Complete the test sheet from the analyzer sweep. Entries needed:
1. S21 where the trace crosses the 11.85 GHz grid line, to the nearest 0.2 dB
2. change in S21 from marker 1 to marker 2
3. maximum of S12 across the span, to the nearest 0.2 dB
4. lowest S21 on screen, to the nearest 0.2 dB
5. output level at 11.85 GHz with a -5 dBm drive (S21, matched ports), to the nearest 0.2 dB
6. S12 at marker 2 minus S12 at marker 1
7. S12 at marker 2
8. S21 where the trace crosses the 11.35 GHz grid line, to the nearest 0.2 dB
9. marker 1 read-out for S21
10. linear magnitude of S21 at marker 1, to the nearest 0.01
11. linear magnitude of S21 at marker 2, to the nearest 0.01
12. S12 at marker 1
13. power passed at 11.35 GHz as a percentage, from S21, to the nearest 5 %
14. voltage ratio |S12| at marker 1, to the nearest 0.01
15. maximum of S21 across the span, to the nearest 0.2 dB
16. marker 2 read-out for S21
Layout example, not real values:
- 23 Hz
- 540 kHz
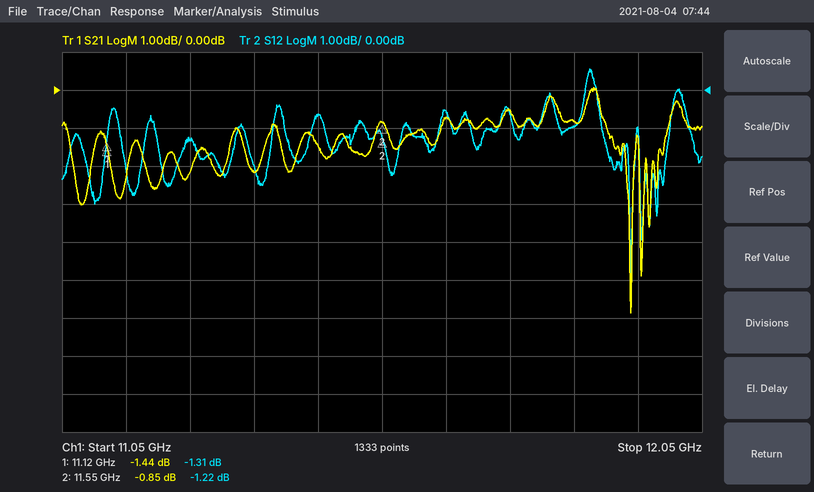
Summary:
- -0.8 dB
- 0.59 dB
- 0.6 dB
- -5.8 dB
- -5.8 dBm
- 0.09 dB
- -1.22 dB
- -2.2 dB
- -1.44 dB
- 0.85
- 0.91
- -1.31 dB
- 60 %
- 0.86
- 0.0 dB
- -0.85 dB
